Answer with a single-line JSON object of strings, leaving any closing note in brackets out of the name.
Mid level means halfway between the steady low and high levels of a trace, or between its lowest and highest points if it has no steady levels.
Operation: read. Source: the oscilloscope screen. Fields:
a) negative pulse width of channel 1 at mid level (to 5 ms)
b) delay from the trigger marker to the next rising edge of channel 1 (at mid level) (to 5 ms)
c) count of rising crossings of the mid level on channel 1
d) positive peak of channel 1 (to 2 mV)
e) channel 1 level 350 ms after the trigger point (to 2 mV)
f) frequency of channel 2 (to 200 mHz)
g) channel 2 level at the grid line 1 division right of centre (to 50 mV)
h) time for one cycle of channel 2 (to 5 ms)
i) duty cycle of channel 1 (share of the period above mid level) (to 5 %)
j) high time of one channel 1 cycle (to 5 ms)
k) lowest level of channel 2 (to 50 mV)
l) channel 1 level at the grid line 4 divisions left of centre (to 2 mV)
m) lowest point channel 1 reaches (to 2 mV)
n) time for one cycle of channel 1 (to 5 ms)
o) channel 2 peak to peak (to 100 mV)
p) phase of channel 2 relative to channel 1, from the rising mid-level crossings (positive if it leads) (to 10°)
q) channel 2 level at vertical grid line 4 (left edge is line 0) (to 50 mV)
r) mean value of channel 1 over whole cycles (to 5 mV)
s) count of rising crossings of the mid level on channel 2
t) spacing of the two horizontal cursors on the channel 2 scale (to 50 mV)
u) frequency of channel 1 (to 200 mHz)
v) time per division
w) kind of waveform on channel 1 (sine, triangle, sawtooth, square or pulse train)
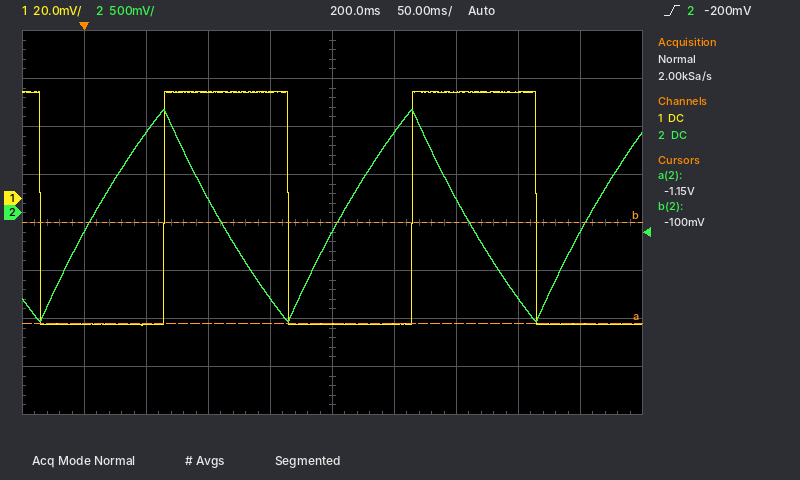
{"negative pulse width of channel 1 at mid level": "100 ms", "delay from the trigger marker to the next rising edge of channel 1 (at mid level)": "65 ms", "count of rising crossings of the mid level on channel 1": "2", "positive peak of channel 1": "44 mV", "channel 1 level 350 ms after the trigger point": "44 mV", "frequency of channel 2": "5.0 Hz", "channel 2 level at the grid line 1 division right of centre": "850 mV", "time for one cycle of channel 2": "200 ms", "duty cycle of channel 1 (share of the period above mid level)": "50 %", "high time of one channel 1 cycle": "100 ms", "lowest level of channel 2": "-1.15 V", "channel 1 level at the grid line 4 divisions left of centre": "-52 mV", "lowest point channel 1 reaches": "-52 mV", "time for one cycle of channel 1": "200 ms", "channel 2 peak to peak": "2.20 V", "phase of channel 2 relative to channel 1, from the rising mid-level crossings (positive if it leads)": "+100°", "channel 2 level at vertical grid line 4 (left edge is line 0)": "-900 mV", "mean value of channel 1 over whole cycles": "-5 mV", "count of rising crossings of the mid level on channel 2": "3", "spacing of the two horizontal cursors on the channel 2 scale": "1.05 V", "frequency of channel 1": "5.0 Hz", "time per division": "50 ms", "kind of waveform on channel 1": "square"}
